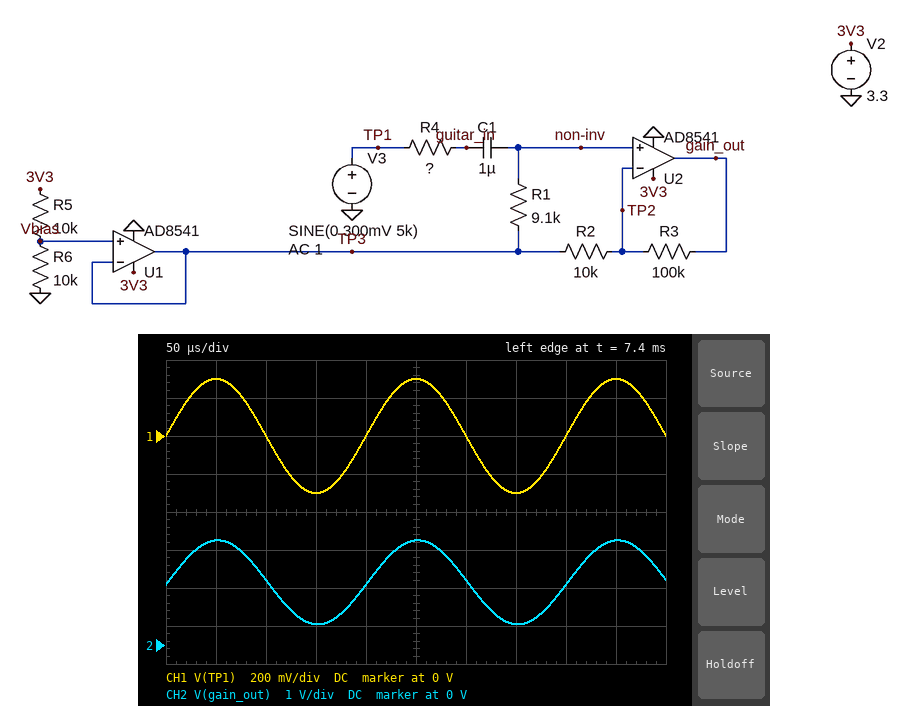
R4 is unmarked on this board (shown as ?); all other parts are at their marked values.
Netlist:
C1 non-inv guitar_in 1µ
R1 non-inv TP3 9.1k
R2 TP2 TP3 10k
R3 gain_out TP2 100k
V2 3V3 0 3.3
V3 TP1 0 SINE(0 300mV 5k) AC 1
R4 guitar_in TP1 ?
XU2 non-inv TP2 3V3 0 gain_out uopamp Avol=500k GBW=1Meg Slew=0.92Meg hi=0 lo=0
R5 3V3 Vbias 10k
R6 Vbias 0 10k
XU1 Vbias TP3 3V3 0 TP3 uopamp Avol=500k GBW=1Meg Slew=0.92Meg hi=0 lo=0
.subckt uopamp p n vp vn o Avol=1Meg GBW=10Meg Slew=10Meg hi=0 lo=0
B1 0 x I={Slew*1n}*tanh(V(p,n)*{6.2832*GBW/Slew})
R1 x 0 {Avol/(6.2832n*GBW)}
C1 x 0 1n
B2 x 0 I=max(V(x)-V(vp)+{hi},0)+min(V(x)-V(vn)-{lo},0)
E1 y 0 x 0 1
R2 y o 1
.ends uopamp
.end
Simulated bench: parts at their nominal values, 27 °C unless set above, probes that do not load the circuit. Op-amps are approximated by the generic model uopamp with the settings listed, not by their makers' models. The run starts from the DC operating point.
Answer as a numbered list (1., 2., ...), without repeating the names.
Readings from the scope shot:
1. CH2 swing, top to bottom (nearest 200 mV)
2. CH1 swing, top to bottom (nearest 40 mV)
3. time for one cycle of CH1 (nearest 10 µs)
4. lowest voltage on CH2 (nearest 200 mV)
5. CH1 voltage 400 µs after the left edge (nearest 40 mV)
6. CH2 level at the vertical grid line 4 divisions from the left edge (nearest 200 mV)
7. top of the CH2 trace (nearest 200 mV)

1. 2.2 V
2. 600 mV
3. 200 µs
4. 600 mV
5. 0 V
6. 1.6 V
7. 2.8 V
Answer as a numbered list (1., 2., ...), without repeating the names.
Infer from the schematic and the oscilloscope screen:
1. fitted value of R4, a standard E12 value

1. 18 kΩ
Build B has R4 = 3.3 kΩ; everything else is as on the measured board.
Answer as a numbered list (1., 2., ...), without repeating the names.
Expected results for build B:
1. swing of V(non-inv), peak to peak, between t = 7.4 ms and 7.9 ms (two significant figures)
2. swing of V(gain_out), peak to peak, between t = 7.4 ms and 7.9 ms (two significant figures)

1. 440 mV
2. 3.3 V
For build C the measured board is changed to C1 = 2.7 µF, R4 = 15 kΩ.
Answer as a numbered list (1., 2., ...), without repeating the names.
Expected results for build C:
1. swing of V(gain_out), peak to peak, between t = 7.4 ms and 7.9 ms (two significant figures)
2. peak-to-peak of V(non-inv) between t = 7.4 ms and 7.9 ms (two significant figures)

1. 2.5 V
2. 230 mV
